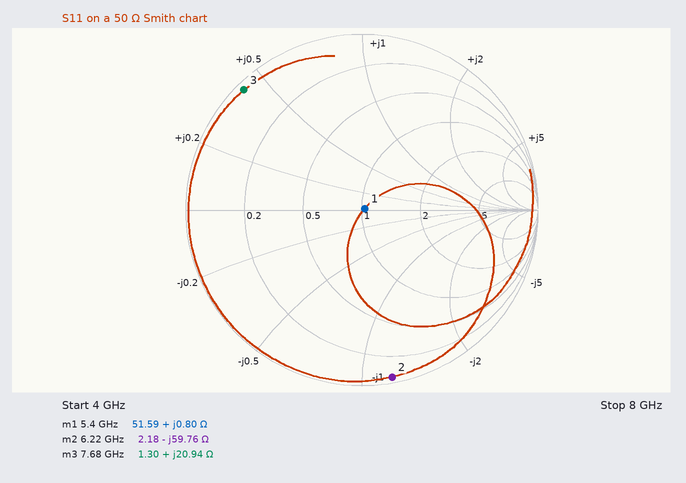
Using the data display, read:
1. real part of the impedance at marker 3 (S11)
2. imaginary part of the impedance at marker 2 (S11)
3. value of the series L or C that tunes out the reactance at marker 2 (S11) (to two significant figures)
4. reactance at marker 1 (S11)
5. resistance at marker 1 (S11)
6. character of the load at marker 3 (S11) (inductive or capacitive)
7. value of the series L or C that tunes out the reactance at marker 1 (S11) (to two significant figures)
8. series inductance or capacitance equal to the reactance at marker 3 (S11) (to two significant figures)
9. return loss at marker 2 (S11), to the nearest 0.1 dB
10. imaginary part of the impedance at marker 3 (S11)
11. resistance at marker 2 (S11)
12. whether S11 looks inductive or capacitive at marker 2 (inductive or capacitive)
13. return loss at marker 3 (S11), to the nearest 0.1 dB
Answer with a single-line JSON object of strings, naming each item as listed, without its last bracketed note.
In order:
{"real part of the impedance at marker 3": "1.30 Ω", "imaginary part of the impedance at marker 2": "-59.76 Ω", "value of the series L or C that tunes out the reactance at marker 2 (S11)": "1.5 nH", "reactance at marker 1": "+0.80 Ω", "resistance at marker 1": "51.59 Ω", "character of the load at marker 3 (S11)": "inductive", "value of the series L or C that tunes out the reactance at marker 1 (S11)": "37 pF", "series inductance or capacitance equal to the reactance at marker 3 (S11)": "430 pH", "return loss at marker 2 (S11), to the nearest 0.1 dB": "0.3 dB", "imaginary part of the impedance at marker 3": "+20.94 Ω", "resistance at marker 2": "2.18 Ω", "whether S11 looks inductive or capacitive at marker 2": "capacitive", "return loss at marker 3 (S11), to the nearest 0.1 dB": "0.4 dB"}
